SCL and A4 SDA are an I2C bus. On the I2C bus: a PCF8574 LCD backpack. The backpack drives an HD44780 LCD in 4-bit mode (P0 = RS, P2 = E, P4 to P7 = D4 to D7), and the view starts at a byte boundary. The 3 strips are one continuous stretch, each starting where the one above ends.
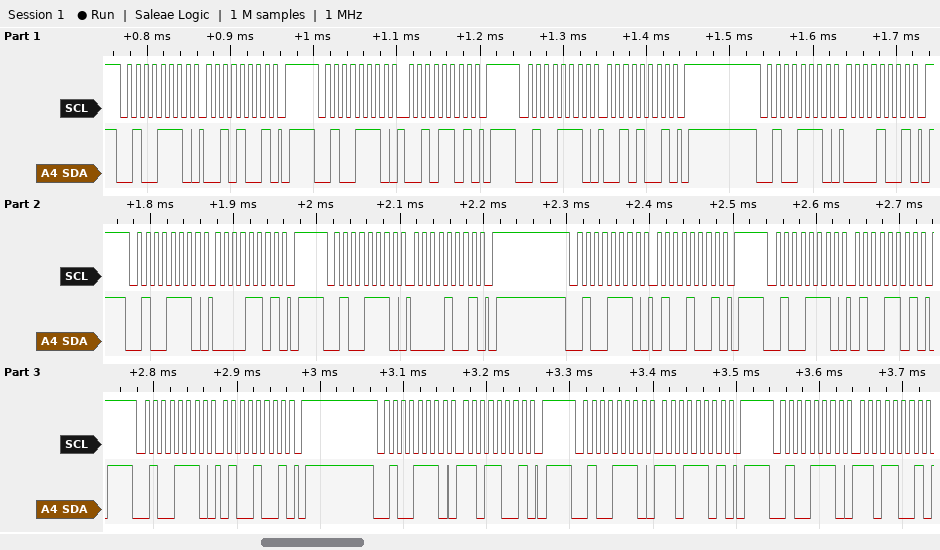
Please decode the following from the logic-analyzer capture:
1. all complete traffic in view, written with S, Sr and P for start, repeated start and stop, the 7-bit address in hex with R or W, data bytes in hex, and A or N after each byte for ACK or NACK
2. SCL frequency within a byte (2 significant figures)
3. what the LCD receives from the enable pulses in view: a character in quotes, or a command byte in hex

S 27W A 29 A P S 27W A 2D A P S 27W A 29 A P S 27W A 09 A P S 27W A 0D A P S 27W A 09 A P S 27W A 49 A P S 27W A 4D A P S 27W A 49 A P S 27W A D9 A P S 27W A DD A P S 27W A D9 A
100 kHz
' ' 'M'
